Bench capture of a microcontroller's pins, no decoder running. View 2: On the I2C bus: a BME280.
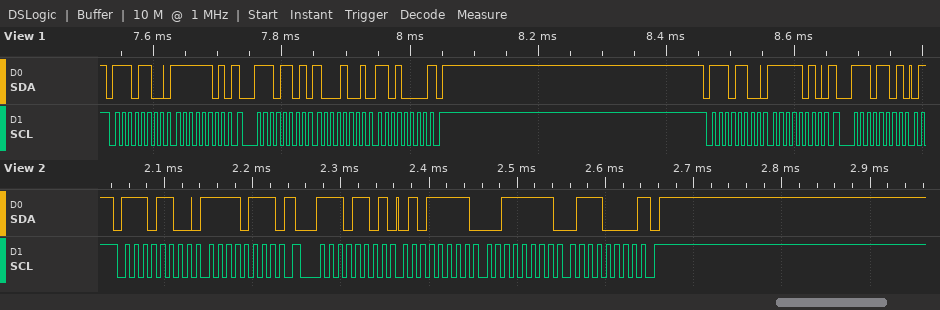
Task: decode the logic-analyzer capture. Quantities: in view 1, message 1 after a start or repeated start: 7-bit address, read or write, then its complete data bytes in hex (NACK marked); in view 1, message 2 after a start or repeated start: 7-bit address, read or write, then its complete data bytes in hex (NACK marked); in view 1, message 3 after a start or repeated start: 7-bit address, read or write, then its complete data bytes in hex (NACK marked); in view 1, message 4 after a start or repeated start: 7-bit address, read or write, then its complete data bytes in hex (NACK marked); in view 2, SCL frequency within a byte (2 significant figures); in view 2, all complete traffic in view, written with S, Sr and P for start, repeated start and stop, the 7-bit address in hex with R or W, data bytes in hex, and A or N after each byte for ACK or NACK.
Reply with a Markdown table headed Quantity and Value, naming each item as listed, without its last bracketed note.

| Quantity | Value |
|---|---|
| in view 1, message 1 after a start or repeated start: 7-bit address, read or write, then its complete data bytes in hex | 0x76 write: FD |
| in view 1, message 2 after a start or repeated start: 7-bit address, read or write, then its complete data bytes in hex | 0x76 read: 89 D0 NACK |
| in view 1, message 3 after a start or repeated start: 7-bit address, read or write, then its complete data bytes in hex | 0x76 write: FA |
| in view 1, message 4 after a start or repeated start: 7-bit address, read or write, then its complete data bytes in hex | 0x76 read |
| in view 2, SCL frequency within a byte | 100 kHz |
| in view 2, all complete traffic in view, written with S, Sr and P for start, repeated start and stop, the 7-bit address in hex with R or W, data bytes in hex, and A or N after each byte for ACK or NACK | S 76W A F7 A Sr 76R A 5F A 3F A 70 N P |
